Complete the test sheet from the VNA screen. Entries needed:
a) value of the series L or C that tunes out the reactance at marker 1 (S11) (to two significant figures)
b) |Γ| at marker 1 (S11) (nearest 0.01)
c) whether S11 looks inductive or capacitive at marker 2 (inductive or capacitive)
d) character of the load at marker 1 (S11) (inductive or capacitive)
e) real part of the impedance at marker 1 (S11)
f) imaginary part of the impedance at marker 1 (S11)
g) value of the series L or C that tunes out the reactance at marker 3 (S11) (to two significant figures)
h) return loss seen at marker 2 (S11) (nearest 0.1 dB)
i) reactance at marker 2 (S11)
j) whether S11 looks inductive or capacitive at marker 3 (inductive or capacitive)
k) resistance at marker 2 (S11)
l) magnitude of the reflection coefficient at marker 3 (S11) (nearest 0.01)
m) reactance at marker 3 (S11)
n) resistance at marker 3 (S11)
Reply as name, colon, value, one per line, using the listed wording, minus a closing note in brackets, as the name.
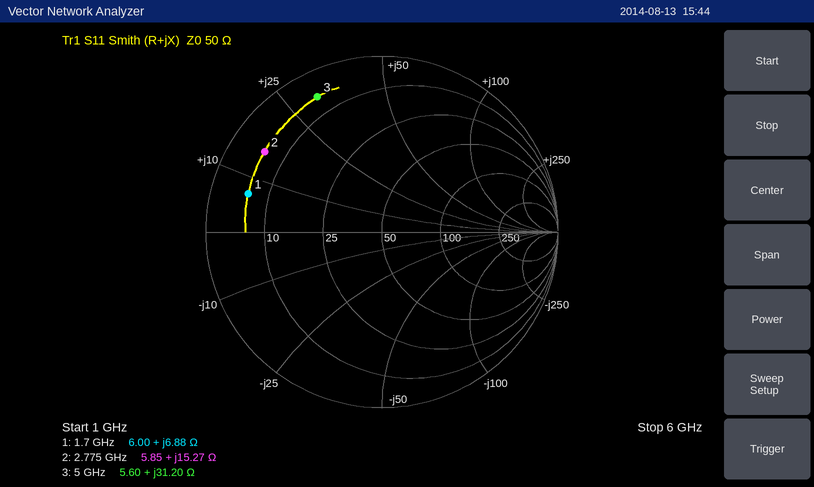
value of the series L or C that tunes out the reactance at marker 1 (S11): 14 pF
|Γ| at marker 1 (S11): 0.79
whether S11 looks inductive or capacitive at marker 2: inductive
character of the load at marker 1 (S11): inductive
real part of the impedance at marker 1: 6.00 Ω
imaginary part of the impedance at marker 1: +6.88 Ω
value of the series L or C that tunes out the reactance at marker 3 (S11): 1.0 pF
return loss seen at marker 2 (S11): 1.9 dB
reactance at marker 2: +15.27 Ω
whether S11 looks inductive or capacitive at marker 3: inductive
resistance at marker 2: 5.85 Ω
magnitude of the reflection coefficient at marker 3 (S11): 0.85
reactance at marker 3: +31.20 Ω
resistance at marker 3: 5.60 Ω
